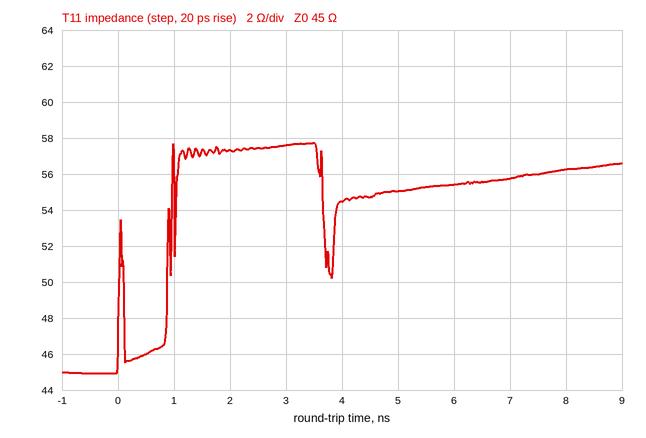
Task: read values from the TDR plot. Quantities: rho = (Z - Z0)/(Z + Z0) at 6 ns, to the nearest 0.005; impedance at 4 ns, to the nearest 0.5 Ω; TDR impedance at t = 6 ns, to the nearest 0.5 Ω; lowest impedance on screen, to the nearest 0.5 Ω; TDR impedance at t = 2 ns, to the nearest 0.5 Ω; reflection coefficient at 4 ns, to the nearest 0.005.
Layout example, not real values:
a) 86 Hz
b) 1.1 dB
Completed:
a) +0.105
b) 54.5 Ω
c) 55.5 Ω
d) 45.0 Ω
e) 57.5 Ω
f) +0.095
